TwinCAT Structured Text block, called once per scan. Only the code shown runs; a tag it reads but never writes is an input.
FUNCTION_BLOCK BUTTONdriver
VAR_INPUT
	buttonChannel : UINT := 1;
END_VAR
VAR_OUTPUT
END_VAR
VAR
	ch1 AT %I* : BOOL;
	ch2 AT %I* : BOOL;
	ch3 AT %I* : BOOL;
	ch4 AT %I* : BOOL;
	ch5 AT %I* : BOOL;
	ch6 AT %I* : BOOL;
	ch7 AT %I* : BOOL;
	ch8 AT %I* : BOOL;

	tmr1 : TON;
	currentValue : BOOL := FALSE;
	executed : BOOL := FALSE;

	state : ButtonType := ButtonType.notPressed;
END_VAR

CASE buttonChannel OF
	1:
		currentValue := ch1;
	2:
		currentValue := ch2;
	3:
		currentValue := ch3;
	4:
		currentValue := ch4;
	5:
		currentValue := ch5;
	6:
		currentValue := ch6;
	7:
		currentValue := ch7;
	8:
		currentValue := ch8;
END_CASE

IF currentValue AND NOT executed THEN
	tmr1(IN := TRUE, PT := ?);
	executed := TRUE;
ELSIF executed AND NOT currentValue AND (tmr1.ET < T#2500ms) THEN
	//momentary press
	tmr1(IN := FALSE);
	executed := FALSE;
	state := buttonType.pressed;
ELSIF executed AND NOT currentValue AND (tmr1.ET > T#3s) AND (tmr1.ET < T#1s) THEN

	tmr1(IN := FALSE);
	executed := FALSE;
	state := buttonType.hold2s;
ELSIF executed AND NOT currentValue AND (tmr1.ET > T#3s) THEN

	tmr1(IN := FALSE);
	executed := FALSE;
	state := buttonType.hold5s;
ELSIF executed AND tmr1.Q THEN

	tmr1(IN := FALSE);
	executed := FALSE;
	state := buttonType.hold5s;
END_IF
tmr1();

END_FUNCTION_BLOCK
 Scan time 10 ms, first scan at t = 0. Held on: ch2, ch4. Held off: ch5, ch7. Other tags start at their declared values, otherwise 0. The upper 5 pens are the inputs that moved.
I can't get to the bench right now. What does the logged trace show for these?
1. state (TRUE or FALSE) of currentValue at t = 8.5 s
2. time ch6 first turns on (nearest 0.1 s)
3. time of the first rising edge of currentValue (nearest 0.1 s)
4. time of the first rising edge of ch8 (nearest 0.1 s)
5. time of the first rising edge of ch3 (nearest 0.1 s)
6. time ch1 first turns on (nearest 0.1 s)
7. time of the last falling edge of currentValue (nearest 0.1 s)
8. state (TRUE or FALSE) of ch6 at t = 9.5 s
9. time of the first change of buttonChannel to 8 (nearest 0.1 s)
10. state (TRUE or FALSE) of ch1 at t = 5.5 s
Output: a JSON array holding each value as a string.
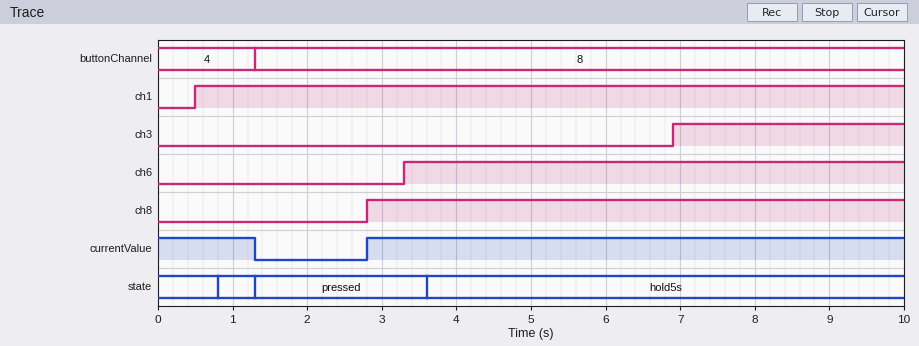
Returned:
["TRUE", "3.3 s", "2.8 s", "2.8 s", "6.9 s", "0.5 s", "1.3 s", "TRUE", "1.3 s", "TRUE"]
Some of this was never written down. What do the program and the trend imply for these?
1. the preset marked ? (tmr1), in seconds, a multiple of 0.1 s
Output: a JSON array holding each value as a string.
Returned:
["0.8 s"]
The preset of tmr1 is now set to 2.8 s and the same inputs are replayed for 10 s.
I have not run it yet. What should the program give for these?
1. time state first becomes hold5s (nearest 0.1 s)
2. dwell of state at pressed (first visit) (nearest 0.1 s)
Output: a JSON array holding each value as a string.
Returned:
["5.6 s", "4.3 s"]
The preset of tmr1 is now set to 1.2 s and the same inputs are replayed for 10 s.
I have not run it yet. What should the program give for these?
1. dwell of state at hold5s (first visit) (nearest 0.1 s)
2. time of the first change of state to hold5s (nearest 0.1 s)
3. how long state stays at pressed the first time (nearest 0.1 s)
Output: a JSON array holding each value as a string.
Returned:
["0.1 s", "1.2 s", "2.7 s"]
